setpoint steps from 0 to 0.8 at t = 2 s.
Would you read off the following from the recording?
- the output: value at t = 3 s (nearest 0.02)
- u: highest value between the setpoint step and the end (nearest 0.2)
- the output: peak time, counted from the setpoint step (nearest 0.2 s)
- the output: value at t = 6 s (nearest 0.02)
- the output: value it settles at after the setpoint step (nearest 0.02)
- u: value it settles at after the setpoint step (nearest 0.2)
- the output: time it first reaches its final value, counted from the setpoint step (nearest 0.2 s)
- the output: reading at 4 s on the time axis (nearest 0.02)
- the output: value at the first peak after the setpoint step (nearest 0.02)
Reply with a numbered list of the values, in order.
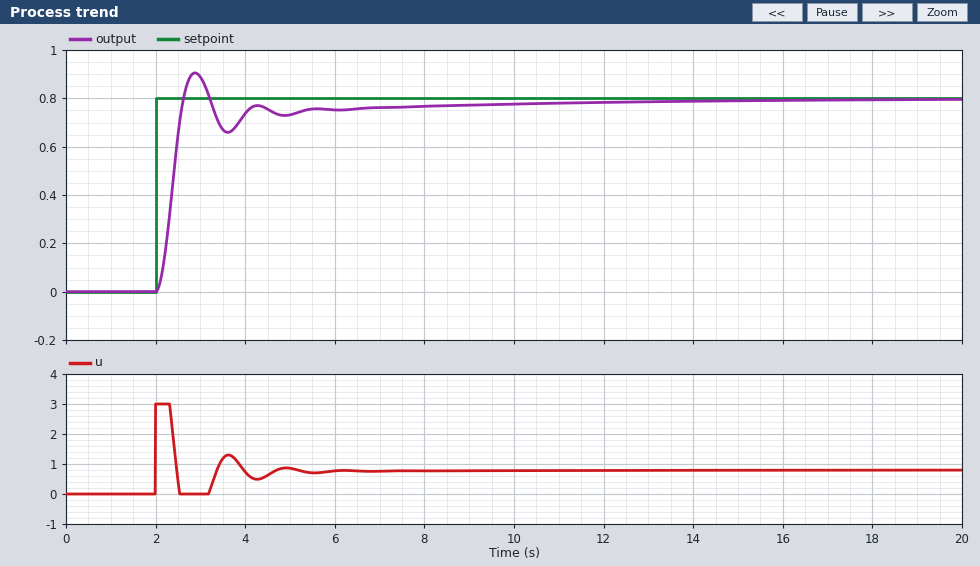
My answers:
1. 0.88
2. 3.0
3. 0.8 s
4. 0.76
5. 0.80
6. 0.8
7. 0.6 s
8. 0.74
9. 0.90
